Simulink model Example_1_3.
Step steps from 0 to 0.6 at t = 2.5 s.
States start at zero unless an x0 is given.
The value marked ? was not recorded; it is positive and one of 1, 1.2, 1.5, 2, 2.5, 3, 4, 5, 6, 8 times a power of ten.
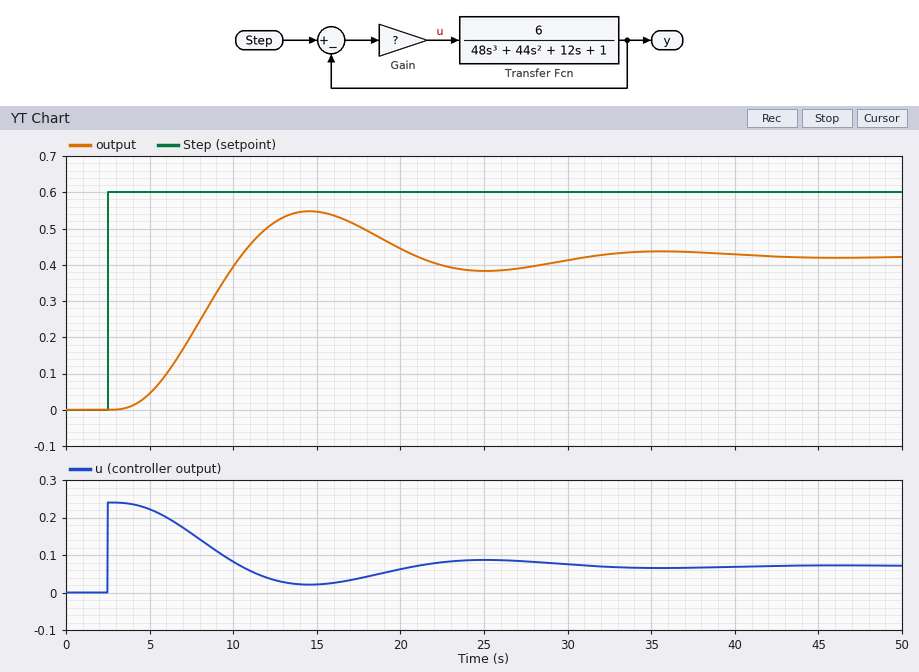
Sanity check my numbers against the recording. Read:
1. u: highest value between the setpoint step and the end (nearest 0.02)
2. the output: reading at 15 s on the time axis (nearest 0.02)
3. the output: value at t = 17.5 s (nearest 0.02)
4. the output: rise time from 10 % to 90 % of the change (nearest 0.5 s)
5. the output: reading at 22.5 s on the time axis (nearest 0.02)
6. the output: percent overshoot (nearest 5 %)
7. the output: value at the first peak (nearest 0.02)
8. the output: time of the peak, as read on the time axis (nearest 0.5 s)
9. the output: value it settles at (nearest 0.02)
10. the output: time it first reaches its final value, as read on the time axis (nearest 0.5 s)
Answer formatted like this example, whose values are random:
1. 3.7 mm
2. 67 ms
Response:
1. 0.24
2. 0.54
3. 0.50
4. 5.0 s
5. 0.40
6. 30 %
7. 0.54
8. 14.5 s
9. 0.42
10. 10.5 s
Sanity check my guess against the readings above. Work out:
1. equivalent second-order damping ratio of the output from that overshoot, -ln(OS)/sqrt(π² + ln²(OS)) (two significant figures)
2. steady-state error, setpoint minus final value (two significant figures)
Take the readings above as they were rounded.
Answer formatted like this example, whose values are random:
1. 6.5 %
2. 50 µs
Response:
1. 0.36
2. 0.18
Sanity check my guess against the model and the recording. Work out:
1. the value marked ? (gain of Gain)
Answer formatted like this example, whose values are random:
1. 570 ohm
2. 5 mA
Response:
1. 0.4
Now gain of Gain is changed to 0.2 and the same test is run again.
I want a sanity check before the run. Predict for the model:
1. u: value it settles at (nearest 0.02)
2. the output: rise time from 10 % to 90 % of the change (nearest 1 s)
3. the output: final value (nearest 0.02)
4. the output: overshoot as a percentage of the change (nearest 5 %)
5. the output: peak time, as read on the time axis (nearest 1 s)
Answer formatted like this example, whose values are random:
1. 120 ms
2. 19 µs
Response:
1. 0.06
2. 7 s
3. 0.32
4. 15 %
5. 18 s
